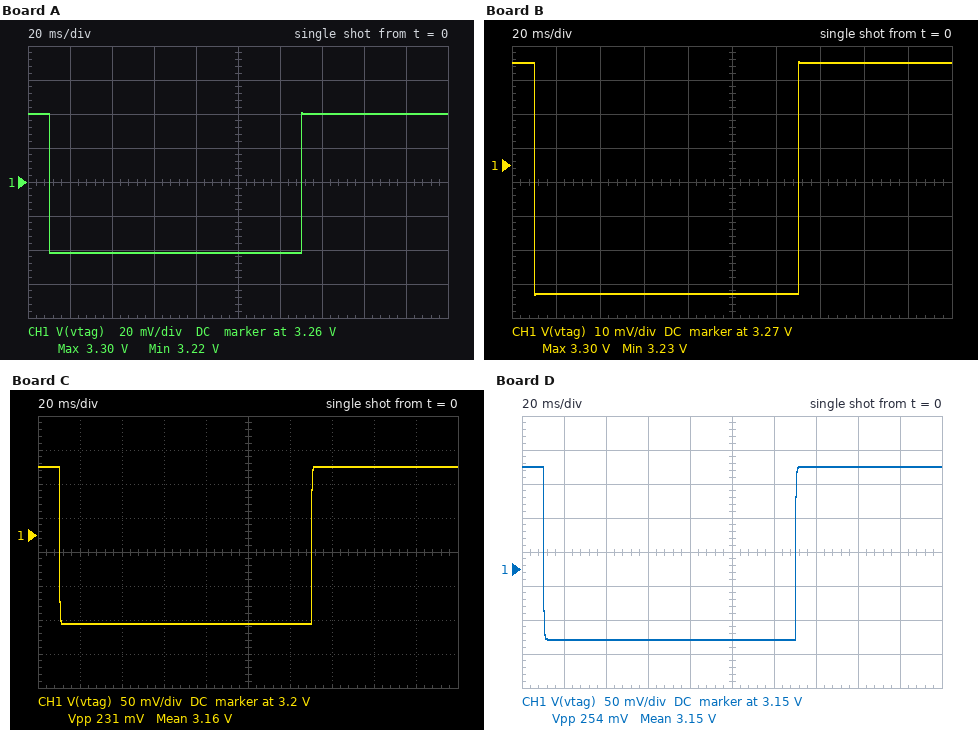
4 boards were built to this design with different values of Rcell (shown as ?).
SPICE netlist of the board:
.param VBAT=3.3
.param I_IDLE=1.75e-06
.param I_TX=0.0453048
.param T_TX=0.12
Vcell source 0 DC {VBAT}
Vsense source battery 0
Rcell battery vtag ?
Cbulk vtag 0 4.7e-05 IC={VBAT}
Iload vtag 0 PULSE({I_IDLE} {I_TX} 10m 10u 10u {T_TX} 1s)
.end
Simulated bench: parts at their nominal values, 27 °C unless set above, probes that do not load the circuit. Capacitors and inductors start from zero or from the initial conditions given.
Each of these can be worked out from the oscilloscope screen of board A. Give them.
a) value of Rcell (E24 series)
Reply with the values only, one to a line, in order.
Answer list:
1.8 Ω
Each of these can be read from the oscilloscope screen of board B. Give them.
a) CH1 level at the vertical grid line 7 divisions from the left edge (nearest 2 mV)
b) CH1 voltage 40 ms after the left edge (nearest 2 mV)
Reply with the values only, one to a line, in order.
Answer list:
3.300 V
3.232 V
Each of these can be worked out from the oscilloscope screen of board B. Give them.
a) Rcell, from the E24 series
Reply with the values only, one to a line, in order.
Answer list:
1.5 Ω
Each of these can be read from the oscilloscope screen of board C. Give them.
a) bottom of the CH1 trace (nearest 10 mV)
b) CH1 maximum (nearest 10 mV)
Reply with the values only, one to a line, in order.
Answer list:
3.07 V
3.30 V
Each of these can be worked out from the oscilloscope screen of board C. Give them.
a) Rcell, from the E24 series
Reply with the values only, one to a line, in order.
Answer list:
5.1 Ω
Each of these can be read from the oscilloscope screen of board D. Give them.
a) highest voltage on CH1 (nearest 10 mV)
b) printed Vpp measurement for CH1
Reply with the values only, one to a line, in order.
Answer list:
3.30 V
254 mV
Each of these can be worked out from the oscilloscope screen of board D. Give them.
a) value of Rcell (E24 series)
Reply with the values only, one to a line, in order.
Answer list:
5.6 Ω
